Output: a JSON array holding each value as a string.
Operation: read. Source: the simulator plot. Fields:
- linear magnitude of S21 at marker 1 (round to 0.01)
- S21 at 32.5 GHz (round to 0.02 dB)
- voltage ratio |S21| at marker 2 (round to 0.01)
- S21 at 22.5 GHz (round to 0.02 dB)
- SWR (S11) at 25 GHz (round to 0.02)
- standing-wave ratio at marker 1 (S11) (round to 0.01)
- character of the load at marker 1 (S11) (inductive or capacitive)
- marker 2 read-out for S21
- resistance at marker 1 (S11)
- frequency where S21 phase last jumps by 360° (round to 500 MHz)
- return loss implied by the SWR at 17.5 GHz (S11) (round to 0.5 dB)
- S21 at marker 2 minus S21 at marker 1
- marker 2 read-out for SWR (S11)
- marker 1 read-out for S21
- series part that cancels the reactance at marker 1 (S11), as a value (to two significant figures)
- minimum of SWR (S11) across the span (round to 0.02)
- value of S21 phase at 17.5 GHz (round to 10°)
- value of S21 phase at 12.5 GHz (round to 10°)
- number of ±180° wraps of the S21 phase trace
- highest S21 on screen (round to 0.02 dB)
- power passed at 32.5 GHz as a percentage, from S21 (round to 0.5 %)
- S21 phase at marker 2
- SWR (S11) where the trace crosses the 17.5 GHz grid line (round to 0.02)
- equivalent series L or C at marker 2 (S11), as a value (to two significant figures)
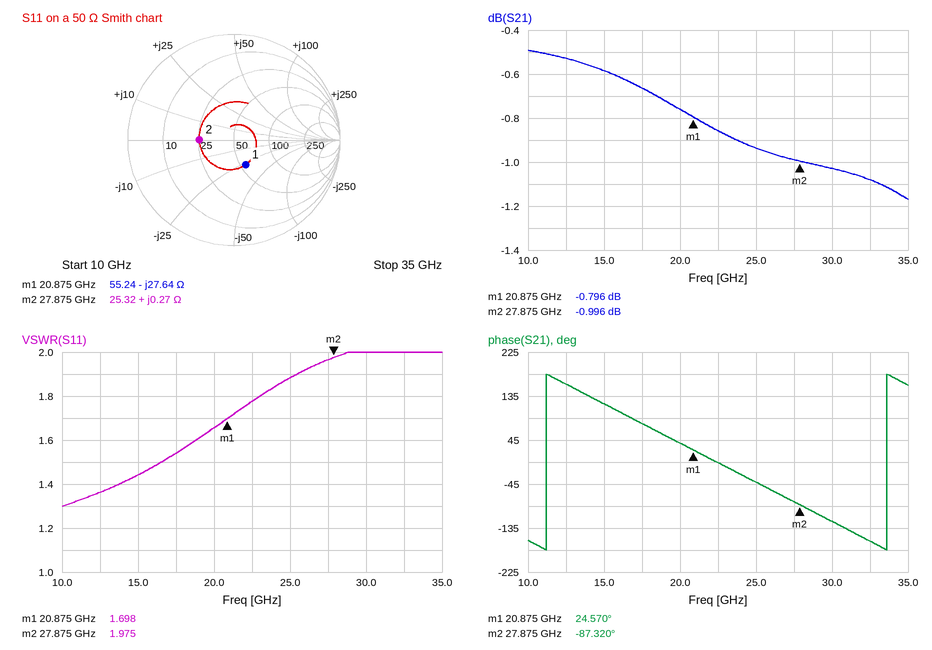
["0.91", "-1.08 dB", "0.89", "-0.86 dB", "1.88", "1.70", "capacitive", "-0.996 dB", "55.24 Ω", "33.5 GHz", "13.5 dB", "-0.200 dB", "1.975", "-0.796 dB", "210 pH", "1.30", "80°", "160°", "2", "-0.50 dB", "78.0 %", "-87.320°", "1.54", "1.5 pH"]
